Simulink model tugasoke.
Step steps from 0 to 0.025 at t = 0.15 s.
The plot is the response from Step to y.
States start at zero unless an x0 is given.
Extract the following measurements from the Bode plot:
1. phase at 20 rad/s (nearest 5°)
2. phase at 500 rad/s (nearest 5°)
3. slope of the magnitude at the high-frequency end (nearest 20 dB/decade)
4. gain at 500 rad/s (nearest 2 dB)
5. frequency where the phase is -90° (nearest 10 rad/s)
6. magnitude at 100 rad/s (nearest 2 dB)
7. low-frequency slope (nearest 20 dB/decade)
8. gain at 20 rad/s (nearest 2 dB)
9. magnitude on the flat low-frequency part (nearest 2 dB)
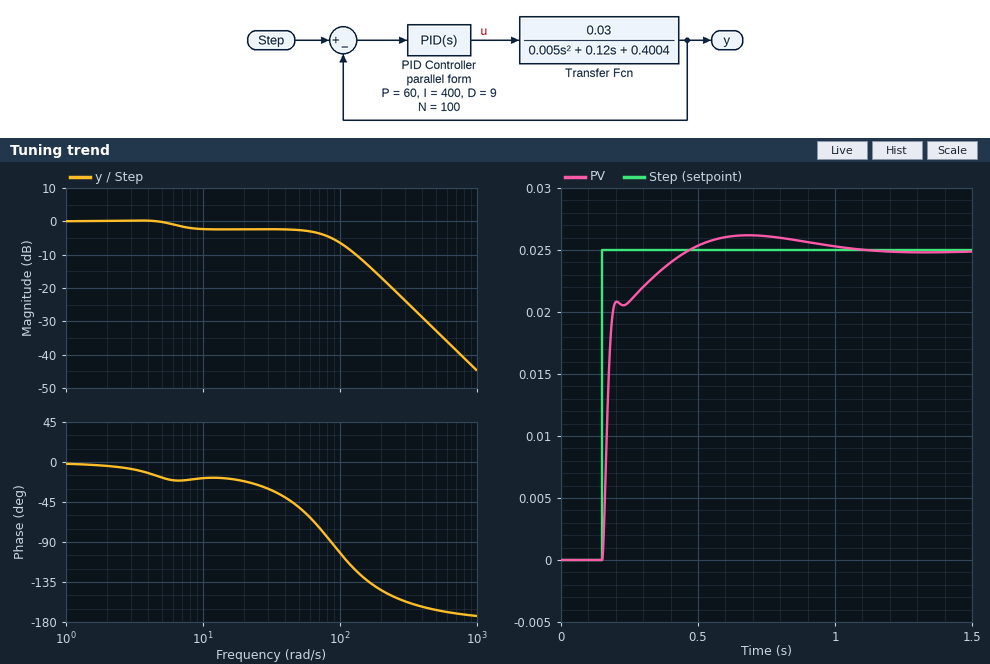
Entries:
-20°
-165°
-40 dB/decade
-32 dB
90 rad/s
-6 dB
0 dB/decade
-2 dB
0 dB
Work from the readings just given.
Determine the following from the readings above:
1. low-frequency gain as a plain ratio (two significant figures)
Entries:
1.0
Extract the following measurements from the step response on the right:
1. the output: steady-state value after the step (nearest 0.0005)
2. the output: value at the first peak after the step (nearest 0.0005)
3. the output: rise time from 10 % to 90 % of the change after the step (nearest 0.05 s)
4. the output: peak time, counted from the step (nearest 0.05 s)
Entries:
0.0250
0.0260
0.15 s
0.55 s
